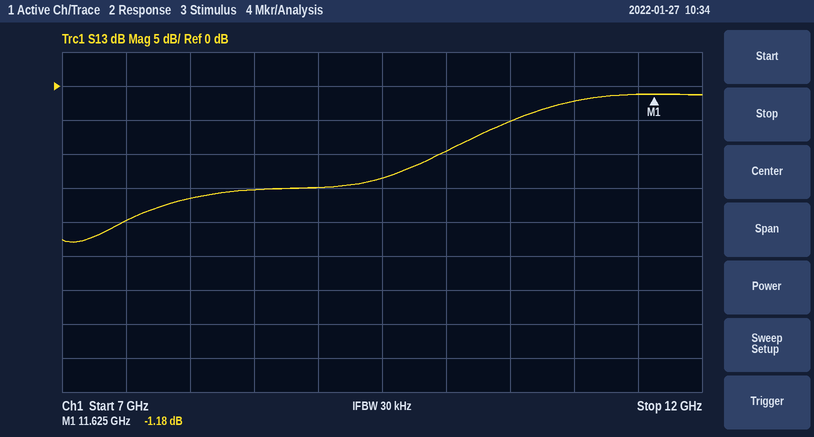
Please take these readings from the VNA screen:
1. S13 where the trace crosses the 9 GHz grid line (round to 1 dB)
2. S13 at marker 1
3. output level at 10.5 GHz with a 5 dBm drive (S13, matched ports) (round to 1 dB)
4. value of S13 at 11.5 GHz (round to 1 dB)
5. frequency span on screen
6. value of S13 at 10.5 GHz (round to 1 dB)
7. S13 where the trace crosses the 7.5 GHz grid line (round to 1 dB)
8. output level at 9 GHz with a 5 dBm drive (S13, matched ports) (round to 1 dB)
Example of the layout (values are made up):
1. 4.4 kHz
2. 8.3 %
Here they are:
1. -15 dB
2. -1.18 dB
3. 0 dBm
4. -1 dB
5. 5 GHz
6. -5 dB
7. -20 dB
8. -10 dBm
